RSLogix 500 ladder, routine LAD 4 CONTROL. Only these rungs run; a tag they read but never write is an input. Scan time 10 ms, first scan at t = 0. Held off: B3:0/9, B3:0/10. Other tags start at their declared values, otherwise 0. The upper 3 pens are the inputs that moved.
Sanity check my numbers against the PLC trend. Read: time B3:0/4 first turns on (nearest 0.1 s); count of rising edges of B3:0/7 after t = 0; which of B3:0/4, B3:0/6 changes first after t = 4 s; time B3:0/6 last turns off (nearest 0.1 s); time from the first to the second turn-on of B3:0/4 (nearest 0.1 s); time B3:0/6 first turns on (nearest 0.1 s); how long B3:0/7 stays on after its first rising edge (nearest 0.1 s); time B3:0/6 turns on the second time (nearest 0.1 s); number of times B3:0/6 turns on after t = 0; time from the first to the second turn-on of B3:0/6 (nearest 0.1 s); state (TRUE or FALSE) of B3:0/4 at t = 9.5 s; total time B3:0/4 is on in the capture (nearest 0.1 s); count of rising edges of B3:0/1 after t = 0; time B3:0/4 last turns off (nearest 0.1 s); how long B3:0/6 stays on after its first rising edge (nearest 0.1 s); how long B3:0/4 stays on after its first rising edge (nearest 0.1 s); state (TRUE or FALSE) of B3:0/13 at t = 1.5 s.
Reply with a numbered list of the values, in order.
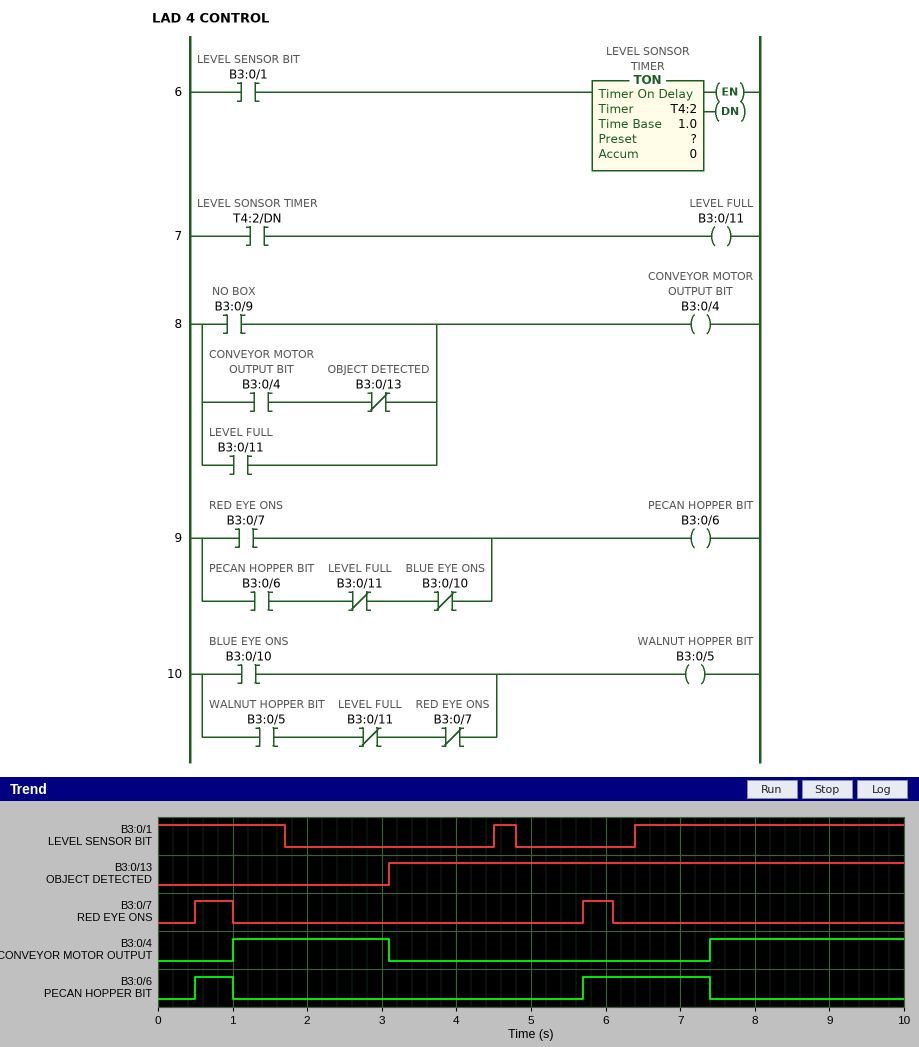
1. 1.0 s
2. 2
3. B3:0/6
4. 7.4 s
5. 6.4 s
6. 0.5 s
7. 0.5 s
8. 5.7 s
9. 2
10. 5.2 s
11. TRUE
12. 4.7 s
13. 2
14. 3.1 s
15. 0.5 s
16. 2.1 s
17. FALSE
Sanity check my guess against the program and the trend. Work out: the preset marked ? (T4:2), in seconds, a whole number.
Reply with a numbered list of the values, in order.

1. 1 s
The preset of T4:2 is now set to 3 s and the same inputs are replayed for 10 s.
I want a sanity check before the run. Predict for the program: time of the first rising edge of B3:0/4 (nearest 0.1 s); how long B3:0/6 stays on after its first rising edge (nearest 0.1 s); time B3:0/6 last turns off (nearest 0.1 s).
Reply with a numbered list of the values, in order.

1. 9.4 s
2. 8.9 s
3. 9.4 s
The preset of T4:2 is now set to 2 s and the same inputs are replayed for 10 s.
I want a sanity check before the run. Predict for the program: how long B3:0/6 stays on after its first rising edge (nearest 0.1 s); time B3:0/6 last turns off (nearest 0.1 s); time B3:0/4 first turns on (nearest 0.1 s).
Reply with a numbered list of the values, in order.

1. 7.9 s
2. 8.4 s
3. 8.4 s
